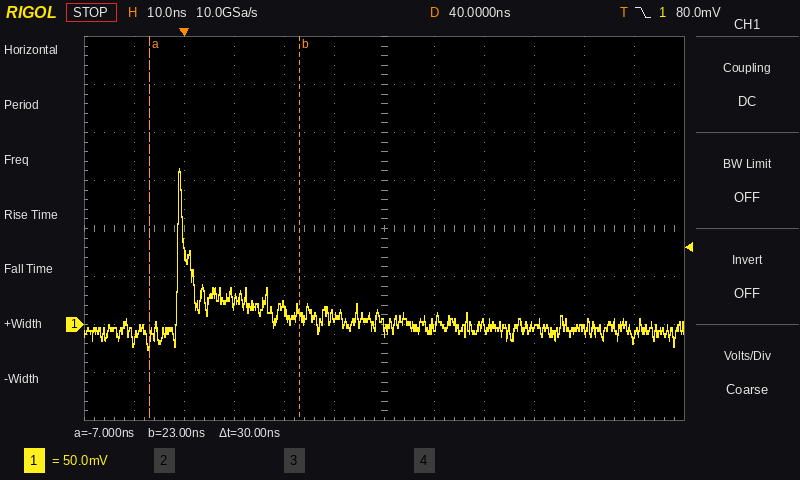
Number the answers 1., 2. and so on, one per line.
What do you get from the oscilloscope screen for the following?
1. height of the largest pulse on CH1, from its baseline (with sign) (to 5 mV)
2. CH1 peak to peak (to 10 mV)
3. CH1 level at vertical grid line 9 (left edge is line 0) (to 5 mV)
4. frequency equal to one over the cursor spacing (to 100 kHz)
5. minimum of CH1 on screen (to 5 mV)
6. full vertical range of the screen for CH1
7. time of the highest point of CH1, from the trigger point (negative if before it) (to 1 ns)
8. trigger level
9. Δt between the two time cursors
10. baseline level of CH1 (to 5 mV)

1. +165 mV
2. 190 mV
3. 0 mV
4. 33.3 MHz
5. -25 mV
6. 400 mV
7. -1 ns
8. 80.0 mV
9. 30 ns
10. -5 mV
